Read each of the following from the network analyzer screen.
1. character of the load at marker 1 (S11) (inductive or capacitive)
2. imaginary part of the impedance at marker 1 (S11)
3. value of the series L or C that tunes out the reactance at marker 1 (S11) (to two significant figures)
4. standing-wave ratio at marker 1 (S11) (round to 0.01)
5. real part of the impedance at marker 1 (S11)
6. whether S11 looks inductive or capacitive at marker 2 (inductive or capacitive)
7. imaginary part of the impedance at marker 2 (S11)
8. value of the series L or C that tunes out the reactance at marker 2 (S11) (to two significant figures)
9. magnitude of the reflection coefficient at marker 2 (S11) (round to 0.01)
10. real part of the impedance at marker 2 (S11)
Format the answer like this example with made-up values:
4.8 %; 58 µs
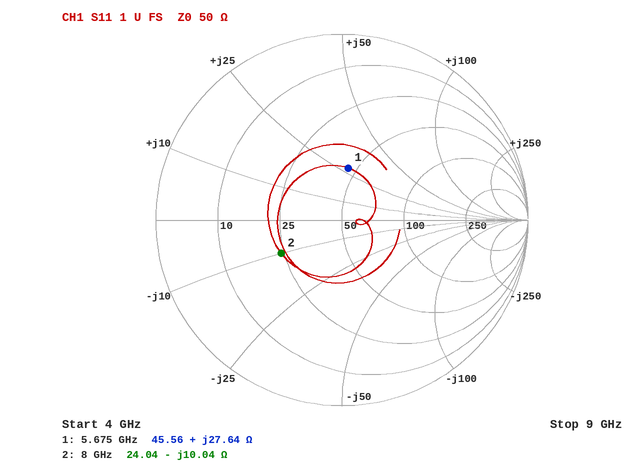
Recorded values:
inductive; +27.64 Ω; 1.0 pF; 1.78; 45.56 Ω; capacitive; -10.04 Ω; 200 pH; 0.37; 24.04 Ω
